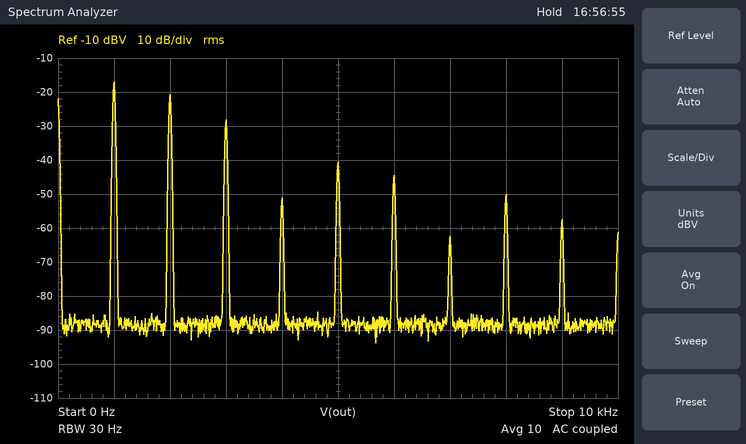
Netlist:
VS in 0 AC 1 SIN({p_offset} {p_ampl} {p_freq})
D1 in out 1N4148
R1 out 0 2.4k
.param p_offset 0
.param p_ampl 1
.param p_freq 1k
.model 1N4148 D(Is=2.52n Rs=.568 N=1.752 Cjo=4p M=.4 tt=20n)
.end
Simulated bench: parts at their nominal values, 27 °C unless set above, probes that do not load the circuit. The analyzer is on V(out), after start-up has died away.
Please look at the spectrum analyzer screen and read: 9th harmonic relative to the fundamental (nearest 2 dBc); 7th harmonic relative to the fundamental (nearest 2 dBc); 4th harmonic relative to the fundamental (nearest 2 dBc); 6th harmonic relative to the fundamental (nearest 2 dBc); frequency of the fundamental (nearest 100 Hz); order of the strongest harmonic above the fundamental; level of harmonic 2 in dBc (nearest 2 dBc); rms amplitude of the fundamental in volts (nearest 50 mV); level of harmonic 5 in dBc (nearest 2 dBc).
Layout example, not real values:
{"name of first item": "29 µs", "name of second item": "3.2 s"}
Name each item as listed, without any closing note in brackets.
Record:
{"9th harmonic relative to the fundamental": "-40 dBc", "7th harmonic relative to the fundamental": "-46 dBc", "4th harmonic relative to the fundamental": "-34 dBc", "6th harmonic relative to the fundamental": "-28 dBc", "frequency of the fundamental": "1.0 kHz", "order of the strongest harmonic above the fundamental": "2", "level of harmonic 2 in dBc": "-4 dBc", "rms amplitude of the fundamental in volts": "150 mV", "level of harmonic 5 in dBc": "-24 dBc"}
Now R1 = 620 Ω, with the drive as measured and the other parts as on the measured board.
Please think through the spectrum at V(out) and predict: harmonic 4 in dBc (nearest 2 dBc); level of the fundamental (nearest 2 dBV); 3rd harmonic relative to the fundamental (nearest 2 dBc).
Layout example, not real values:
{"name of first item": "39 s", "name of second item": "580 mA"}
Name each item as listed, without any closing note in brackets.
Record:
{"harmonic 4 in dBc": "-24 dBc", "level of the fundamental": "-18 dBV", "3rd harmonic relative to the fundamental": "-10 dBc"}
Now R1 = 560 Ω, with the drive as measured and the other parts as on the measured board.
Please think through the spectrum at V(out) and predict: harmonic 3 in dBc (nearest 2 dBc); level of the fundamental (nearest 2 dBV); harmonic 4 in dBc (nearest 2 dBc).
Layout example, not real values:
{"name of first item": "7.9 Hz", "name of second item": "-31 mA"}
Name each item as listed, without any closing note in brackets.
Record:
{"harmonic 3 in dBc": "-10 dBc", "level of the fundamental": "-18 dBV", "harmonic 4 in dBc": "-24 dBc"}
